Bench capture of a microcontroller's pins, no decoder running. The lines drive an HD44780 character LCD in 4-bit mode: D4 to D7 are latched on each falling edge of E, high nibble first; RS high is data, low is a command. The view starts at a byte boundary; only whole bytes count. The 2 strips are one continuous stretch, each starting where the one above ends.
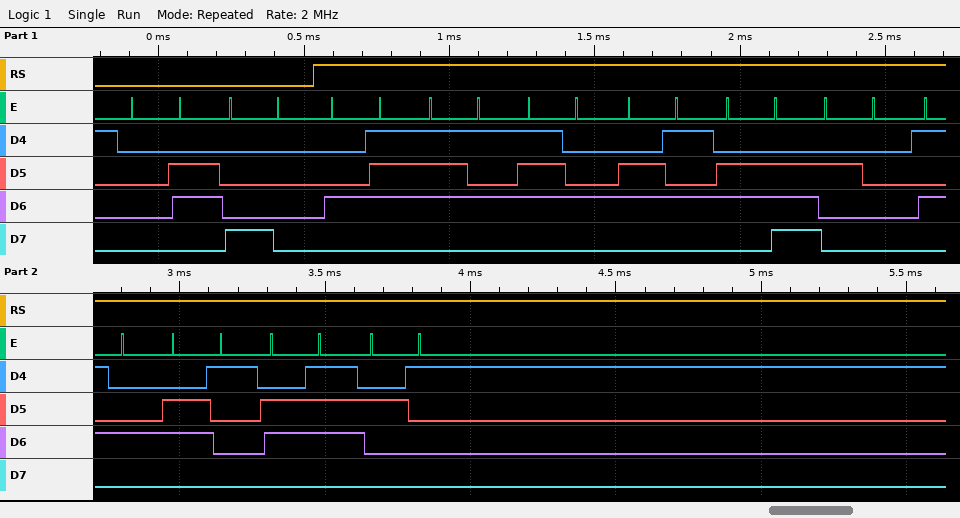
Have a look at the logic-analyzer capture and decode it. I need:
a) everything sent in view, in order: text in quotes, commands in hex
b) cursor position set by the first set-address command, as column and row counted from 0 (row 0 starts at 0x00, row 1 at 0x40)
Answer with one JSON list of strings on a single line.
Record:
["0x06 0x80 \"Guten Tag!\"", "column 0, row 0"]
